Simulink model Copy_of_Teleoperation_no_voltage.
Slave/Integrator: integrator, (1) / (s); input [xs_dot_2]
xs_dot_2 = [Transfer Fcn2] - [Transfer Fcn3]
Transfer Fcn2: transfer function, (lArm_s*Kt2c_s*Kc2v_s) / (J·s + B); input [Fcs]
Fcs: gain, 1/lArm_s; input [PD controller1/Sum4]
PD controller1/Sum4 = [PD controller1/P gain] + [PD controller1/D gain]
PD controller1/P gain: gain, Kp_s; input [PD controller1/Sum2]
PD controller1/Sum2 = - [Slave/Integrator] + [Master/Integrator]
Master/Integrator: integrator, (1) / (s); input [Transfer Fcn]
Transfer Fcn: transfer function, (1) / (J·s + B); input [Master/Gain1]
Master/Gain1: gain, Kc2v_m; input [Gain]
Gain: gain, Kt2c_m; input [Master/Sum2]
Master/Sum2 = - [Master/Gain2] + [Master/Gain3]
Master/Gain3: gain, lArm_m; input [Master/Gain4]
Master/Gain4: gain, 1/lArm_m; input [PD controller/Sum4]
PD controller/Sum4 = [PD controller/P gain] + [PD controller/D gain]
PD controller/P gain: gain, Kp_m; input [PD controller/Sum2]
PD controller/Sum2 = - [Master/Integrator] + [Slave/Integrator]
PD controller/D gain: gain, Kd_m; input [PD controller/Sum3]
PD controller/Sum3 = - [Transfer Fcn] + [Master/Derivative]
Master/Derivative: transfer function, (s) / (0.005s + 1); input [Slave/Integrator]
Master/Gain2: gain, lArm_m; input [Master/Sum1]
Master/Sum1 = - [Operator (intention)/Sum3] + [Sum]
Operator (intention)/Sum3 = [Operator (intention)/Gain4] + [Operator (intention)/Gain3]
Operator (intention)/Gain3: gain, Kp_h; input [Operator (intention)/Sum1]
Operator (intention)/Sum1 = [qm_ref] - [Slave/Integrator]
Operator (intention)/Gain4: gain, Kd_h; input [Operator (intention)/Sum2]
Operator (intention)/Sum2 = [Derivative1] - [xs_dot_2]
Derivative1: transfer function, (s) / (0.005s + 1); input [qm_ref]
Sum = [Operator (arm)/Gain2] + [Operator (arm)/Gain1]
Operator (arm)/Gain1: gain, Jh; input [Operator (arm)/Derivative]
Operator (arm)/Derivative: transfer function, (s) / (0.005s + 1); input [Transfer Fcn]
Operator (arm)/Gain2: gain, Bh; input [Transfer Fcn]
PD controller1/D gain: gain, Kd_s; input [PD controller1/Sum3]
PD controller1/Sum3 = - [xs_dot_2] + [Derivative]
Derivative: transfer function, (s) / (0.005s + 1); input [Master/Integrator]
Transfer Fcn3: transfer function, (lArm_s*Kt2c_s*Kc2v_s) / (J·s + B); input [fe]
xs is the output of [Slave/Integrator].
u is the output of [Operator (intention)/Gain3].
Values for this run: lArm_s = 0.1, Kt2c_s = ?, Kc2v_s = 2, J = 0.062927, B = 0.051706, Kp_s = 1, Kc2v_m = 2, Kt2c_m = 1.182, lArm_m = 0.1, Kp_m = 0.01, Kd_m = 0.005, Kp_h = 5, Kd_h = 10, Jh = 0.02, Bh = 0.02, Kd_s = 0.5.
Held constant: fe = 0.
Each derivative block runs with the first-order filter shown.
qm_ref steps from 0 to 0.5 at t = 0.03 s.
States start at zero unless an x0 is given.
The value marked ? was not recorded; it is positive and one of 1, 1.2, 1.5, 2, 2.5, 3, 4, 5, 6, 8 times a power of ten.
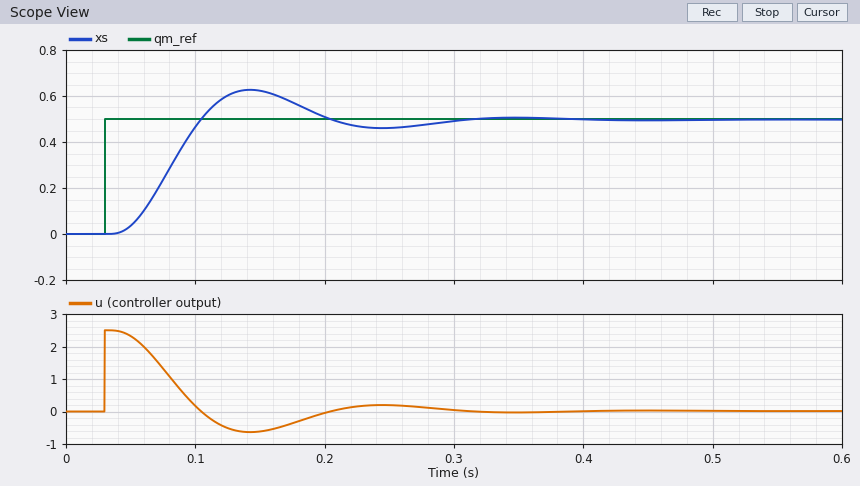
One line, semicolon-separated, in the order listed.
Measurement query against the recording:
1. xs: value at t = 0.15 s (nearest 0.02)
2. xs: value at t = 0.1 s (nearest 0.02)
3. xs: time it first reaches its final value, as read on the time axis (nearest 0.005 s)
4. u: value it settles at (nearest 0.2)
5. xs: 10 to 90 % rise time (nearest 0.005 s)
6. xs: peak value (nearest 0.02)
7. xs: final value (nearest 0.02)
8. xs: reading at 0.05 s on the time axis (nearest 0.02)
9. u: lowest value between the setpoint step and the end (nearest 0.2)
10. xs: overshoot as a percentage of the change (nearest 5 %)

0.62; 0.46; 0.105 s; 0.0; 0.045 s; 0.62; 0.50; 0.04; -0.6; 25 %
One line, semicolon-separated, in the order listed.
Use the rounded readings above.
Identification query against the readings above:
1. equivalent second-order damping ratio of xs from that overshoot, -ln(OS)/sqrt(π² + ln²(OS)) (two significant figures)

0.40
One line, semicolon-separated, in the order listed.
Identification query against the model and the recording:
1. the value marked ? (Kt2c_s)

2
